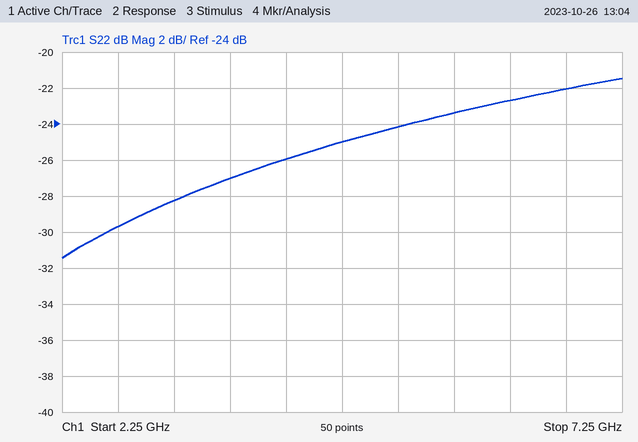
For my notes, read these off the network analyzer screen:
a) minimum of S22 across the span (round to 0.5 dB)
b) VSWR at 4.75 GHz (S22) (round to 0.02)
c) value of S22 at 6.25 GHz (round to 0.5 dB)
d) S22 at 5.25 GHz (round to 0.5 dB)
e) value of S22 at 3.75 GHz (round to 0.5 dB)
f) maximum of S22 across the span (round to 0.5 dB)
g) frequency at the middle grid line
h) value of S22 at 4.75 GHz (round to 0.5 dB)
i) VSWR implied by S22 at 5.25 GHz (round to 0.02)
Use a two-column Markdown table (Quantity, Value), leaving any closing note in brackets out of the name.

| Quantity | Value |
|---|---|
| minimum of S22 across the span | -31.5 dB |
| VSWR at 4.75 GHz (S22) | 1.12 |
| value of S22 at 6.25 GHz | -22.5 dB |
| S22 at 5.25 GHz | -24.0 dB |
| value of S22 at 3.75 GHz | -27.0 dB |
| maximum of S22 across the span | -21.5 dB |
| frequency at the middle grid line | 4.75 GHz |
| value of S22 at 4.75 GHz | -25.0 dB |
| VSWR implied by S22 at 5.25 GHz | 1.14 |
